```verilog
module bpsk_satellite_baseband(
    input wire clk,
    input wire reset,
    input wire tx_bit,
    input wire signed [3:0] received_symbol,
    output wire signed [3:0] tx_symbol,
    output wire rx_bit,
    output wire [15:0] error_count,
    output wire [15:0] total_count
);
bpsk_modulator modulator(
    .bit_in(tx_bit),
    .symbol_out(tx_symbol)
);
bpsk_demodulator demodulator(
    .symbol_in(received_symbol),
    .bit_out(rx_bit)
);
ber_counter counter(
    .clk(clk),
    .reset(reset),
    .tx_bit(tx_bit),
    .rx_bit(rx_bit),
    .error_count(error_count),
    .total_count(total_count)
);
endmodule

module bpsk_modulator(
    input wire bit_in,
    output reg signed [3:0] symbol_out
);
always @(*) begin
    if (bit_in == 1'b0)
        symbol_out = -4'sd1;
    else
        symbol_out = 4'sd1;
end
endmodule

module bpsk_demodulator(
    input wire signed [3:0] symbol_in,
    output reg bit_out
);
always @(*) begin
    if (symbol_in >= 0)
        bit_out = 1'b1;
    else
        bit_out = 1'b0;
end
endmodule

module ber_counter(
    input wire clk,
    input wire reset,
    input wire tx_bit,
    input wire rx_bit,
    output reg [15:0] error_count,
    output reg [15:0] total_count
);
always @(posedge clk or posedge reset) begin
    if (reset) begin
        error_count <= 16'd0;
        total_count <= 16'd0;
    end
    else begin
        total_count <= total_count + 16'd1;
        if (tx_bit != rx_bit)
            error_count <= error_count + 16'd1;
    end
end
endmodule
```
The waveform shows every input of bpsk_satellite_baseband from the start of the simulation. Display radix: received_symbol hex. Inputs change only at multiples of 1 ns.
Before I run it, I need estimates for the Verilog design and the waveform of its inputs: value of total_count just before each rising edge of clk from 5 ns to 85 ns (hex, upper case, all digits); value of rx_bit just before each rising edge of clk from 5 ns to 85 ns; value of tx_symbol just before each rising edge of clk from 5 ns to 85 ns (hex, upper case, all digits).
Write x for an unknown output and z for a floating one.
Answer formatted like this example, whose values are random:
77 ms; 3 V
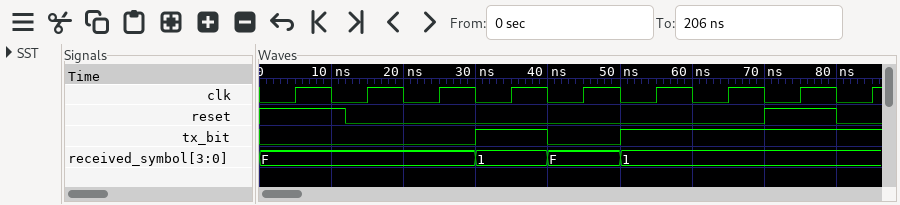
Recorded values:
0000, 0000, 0001, 0002, 0003, 0004, 0005, 0000, 0000; 0 0 0 1 0 1 1 1 1; F, F, F, 1, F, 1, 1, 1, 1
